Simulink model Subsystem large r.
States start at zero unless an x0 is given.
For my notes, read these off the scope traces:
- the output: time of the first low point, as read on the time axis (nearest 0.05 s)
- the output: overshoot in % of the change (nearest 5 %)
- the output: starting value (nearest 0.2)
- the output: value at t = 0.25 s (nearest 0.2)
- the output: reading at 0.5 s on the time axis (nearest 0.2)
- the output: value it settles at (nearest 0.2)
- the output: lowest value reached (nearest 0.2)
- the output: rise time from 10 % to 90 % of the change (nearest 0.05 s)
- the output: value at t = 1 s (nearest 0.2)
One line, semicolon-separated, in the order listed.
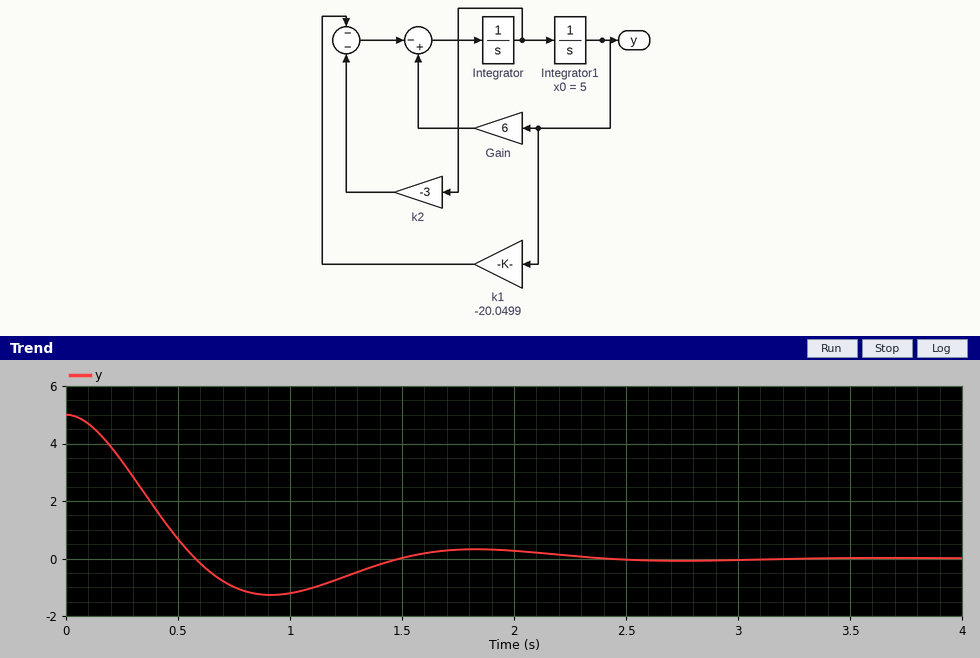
0.90 s; 25 %; 5.0; 3.4; 0.6; 0.0; -1.2; 0.40 s; -1.2
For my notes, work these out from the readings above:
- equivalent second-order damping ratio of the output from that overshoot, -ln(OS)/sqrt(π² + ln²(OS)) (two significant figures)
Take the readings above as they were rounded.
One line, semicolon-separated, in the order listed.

0.40
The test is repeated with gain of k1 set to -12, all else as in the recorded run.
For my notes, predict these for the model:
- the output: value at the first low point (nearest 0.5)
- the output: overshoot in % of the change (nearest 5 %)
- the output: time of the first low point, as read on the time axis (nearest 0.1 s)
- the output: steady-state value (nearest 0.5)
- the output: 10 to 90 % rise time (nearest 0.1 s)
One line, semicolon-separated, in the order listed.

-0.5; 10 %; 1.6 s; 0.0; 0.8 s
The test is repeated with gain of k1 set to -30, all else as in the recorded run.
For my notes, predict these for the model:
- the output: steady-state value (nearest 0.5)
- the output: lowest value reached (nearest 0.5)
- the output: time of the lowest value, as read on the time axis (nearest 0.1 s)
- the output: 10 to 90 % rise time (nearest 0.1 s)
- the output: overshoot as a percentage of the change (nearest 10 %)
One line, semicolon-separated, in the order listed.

0.0; -2.0; 0.7 s; 0.3 s; 40 %
